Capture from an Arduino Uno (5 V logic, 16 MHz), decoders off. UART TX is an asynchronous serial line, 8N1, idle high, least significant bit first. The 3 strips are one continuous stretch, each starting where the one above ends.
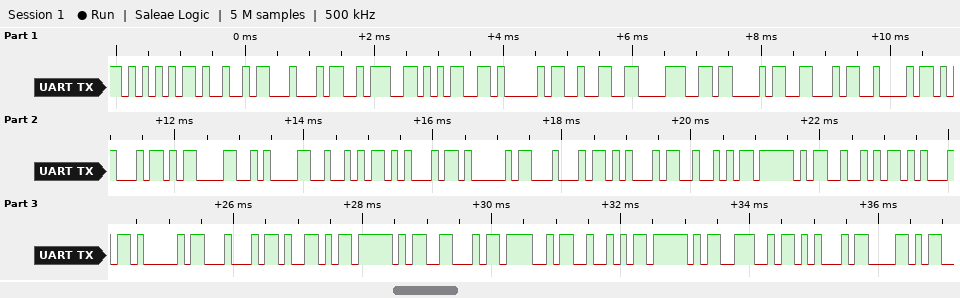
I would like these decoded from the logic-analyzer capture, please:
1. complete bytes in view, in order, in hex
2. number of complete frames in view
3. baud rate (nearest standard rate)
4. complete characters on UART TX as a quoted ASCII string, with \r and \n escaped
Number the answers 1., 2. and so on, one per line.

1. 55 49 44 3A 35 41 32 38 43 46 42 45 0D 0A 52 45 41 44 45 52 5F 52 45 41 44 59 5F 46 4F 52 5F 4E 45 58
2. 34
3. 9600 baud
4. "UID:5A28CFBE\r\nREADER_READY_FOR_NEX"
